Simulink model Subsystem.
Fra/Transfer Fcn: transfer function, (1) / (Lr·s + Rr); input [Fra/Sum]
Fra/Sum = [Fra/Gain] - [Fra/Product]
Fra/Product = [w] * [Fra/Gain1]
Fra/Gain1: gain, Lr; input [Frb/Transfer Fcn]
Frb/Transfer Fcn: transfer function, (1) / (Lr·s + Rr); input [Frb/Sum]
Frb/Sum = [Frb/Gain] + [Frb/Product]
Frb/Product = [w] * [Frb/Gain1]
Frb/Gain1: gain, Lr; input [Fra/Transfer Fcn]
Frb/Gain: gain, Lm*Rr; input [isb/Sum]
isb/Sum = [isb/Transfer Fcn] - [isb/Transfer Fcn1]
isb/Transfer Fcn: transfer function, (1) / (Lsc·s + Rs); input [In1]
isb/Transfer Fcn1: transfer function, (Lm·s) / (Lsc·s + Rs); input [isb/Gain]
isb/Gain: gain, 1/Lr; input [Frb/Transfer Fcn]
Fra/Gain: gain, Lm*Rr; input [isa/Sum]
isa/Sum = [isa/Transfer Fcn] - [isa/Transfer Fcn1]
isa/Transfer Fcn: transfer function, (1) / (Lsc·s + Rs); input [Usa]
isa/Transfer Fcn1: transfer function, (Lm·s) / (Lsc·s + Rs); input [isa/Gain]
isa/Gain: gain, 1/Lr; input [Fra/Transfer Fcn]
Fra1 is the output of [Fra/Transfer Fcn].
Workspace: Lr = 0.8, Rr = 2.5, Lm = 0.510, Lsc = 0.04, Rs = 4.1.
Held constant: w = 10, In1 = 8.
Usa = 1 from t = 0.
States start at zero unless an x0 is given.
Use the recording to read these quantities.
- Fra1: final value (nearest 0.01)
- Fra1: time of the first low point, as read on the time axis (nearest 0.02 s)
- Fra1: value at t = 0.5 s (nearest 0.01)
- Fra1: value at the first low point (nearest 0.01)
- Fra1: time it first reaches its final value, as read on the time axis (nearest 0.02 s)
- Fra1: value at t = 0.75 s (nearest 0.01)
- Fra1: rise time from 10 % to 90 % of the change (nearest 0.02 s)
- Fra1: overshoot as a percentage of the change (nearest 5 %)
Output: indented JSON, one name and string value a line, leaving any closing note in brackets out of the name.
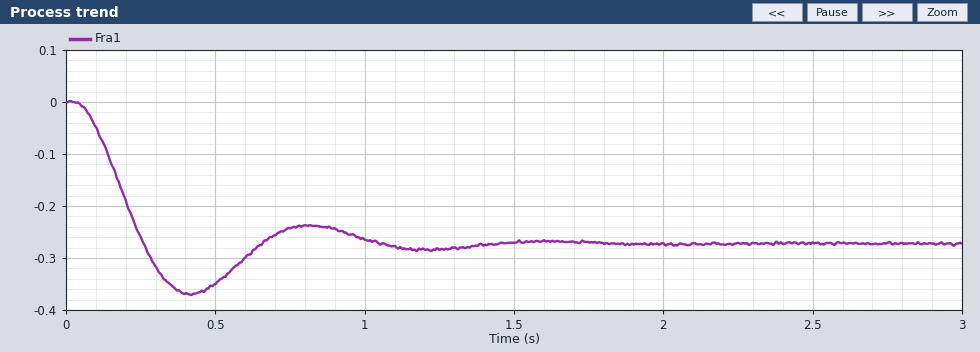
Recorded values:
{
  "Fra1: final value": "-0.27",
  "Fra1: time of the first low point, as read on the time axis": "0.42 s",
  "Fra1: value at t = 0.5 s": "-0.35",
  "Fra1: value at the first low point": "-0.37",
  "Fra1: time it first reaches its final value, as read on the time axis": "0.26 s",
  "Fra1: value at t = 0.75 s": "-0.24",
  "Fra1: rise time from 10 % to 90 % of the change": "0.16 s",
  "Fra1: overshoot as a percentage of the change": "35 %"
}
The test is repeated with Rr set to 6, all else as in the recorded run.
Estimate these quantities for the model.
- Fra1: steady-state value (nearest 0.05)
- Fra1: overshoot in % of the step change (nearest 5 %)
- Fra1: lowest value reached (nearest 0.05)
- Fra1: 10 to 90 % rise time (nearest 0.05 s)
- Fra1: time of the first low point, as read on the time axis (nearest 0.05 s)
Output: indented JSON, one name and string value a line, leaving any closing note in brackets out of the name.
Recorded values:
{
  "Fra1: steady-state value": "-0.45",
  "Fra1: overshoot in % of the step change": "10 %",
  "Fra1: lowest value reached": "-0.45",
  "Fra1: 10 to 90 % rise time": "0.25 s",
  "Fra1: time of the first low point, as read on the time axis": "0.55 s"
}
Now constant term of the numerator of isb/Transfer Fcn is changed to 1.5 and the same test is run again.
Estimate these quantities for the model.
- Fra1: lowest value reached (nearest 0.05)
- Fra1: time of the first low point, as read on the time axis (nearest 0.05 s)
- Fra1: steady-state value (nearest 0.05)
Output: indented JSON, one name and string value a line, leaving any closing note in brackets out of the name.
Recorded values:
{
  "Fra1: lowest value reached": "-0.55",
  "Fra1: time of the first low point, as read on the time axis": "0.40 s",
  "Fra1: steady-state value": "-0.40"
}
